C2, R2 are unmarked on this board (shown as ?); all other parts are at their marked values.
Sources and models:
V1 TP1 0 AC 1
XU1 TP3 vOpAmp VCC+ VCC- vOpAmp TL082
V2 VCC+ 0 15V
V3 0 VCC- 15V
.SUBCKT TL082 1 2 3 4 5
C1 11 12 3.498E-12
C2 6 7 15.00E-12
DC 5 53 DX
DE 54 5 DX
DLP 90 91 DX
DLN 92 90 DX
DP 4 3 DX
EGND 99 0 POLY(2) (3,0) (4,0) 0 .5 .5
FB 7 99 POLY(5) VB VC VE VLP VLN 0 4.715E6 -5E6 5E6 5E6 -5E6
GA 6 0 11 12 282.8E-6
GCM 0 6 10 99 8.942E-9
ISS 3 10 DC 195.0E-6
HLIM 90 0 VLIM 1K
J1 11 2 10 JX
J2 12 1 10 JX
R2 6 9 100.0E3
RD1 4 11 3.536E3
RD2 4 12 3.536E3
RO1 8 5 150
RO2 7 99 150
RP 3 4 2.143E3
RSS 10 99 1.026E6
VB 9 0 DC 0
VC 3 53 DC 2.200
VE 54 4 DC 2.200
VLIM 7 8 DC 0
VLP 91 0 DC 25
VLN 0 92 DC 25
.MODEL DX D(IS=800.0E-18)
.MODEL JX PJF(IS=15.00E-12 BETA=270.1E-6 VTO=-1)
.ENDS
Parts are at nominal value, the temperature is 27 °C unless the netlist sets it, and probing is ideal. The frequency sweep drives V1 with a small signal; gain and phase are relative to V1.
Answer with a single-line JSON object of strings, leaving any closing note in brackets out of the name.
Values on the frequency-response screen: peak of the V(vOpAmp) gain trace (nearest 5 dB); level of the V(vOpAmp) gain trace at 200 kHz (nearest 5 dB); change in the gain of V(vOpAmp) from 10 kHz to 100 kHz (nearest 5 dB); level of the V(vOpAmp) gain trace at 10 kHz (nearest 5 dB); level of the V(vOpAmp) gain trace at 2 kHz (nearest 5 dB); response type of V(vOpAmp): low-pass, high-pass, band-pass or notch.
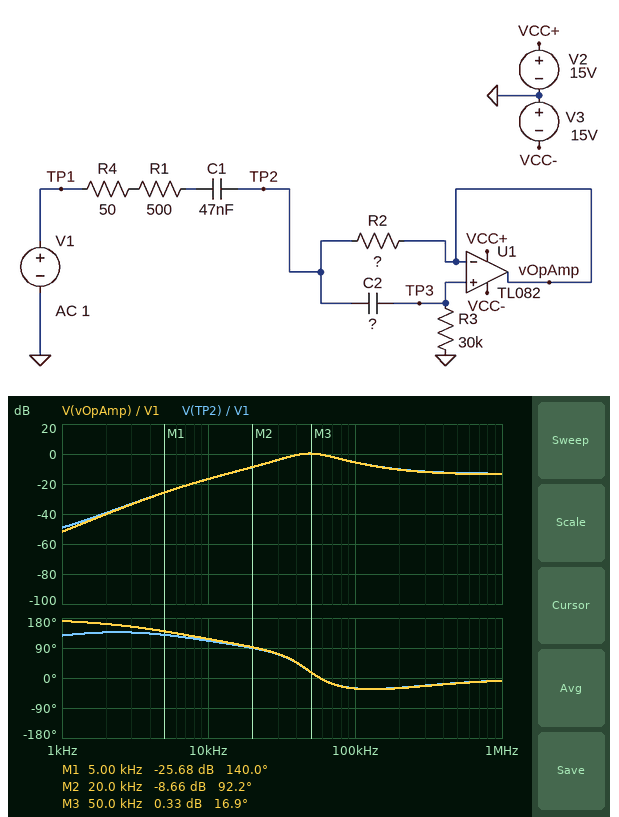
{"peak of the V(vOpAmp) gain trace": "0 dB", "level of the V(vOpAmp) gain trace at 200 kHz": "-10 dB", "change in the gain of V(vOpAmp) from 10 kHz to 100 kHz": "10 dB", "level of the V(vOpAmp) gain trace at 10 kHz": "-15 dB", "level of the V(vOpAmp) gain trace at 2 kHz": "-40 dB", "response type of V(vOpAmp): low-pass, high-pass, band-pass or notch": "band-pass"}
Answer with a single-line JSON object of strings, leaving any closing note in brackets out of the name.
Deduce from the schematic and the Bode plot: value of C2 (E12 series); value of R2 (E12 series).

{"value of C2": "5.6 nF", "value of R2": "8.2 Ω"}
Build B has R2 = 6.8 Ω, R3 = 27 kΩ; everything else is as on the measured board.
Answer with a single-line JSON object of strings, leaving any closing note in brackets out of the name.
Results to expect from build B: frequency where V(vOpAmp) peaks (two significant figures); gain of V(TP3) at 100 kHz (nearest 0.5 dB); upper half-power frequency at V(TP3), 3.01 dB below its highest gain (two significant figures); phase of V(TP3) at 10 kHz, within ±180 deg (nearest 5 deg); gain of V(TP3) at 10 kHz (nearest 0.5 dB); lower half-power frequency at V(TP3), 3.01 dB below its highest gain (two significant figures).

{"frequency where V(vOpAmp) peaks": "52 kHz", "gain of V(TP3) at 100 kHz": "-6.0 dB", "upper half-power frequency at V(TP3), 3.01 dB below its highest gain": "73 kHz", "phase of V(TP3) at 10 kHz, within ±180 deg": "120 deg", "gain of V(TP3) at 10 kHz": "-19.5 dB", "lower half-power frequency at V(TP3), 3.01 dB below its highest gain": "38 kHz"}
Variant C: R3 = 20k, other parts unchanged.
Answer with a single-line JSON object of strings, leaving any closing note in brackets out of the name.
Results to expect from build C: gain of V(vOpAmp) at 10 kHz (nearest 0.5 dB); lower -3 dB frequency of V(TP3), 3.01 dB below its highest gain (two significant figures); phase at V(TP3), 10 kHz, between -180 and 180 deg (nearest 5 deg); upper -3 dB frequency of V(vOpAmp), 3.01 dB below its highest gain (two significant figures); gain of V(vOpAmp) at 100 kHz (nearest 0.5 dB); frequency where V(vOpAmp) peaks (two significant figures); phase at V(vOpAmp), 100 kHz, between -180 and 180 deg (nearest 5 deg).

{"gain of V(vOpAmp) at 10 kHz": "-20.5 dB", "lower -3 dB frequency of V(TP3), 3.01 dB below its highest gain": "44 kHz", "phase at V(TP3), 10 kHz, between -180 and 180 deg": "120 deg", "upper -3 dB frequency of V(vOpAmp), 3.01 dB below its highest gain": "86 kHz", "gain of V(vOpAmp) at 100 kHz": "-4.5 dB", "frequency where V(vOpAmp) peaks": "61 kHz", "phase at V(vOpAmp), 100 kHz, between -180 and 180 deg": "-25 deg"}
